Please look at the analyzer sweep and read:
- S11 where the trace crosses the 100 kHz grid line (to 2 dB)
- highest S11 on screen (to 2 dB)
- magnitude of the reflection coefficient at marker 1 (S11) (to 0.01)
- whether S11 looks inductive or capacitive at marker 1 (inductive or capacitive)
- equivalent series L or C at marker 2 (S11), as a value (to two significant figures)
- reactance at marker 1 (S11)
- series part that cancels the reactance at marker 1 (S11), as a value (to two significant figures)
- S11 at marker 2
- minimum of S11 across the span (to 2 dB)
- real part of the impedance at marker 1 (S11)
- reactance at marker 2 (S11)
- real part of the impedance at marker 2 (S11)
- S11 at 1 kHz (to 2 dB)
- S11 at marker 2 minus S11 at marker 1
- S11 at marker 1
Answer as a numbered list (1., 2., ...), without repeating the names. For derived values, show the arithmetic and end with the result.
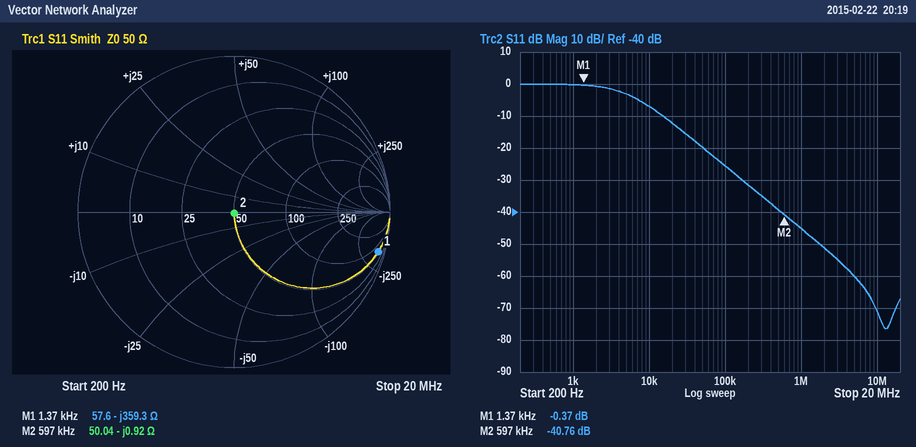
1. -26 dB
2. 0 dB
3. 0.96
4. capacitive
5. C = 1/(2π × 597 kHz × 0.92 Ω) ≈ 290 nF
6. -359.3 Ω
7. L = 359.3 Ω/(2π × 1.37 kHz) ≈ 42 mH
8. -40.76 dB
9. -76 dB
10. 57.6 Ω
11. -0.92 Ω
12. 50.04 Ω
13. 0 dB
14. -40.76 − (-0.37) = -40.39 dB
15. -0.37 dB
